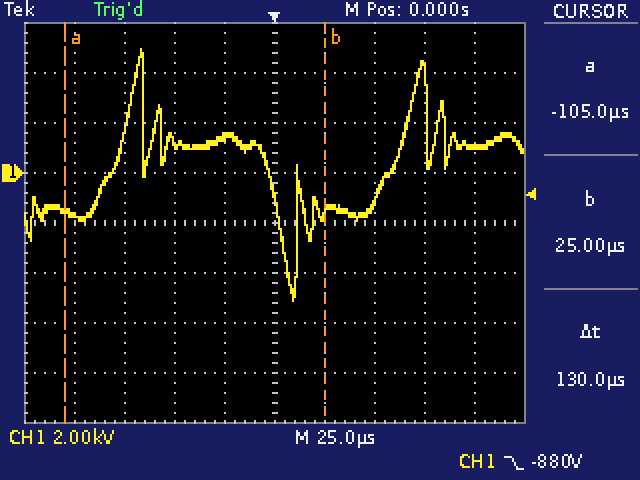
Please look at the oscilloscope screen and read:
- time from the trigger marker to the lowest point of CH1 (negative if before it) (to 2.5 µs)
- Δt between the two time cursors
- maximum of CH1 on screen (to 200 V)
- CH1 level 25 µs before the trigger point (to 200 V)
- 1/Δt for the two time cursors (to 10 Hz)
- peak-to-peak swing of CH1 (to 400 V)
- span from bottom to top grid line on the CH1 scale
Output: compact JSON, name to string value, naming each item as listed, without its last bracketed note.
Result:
{"time from the trigger marker to the lowest point of CH1 (negative if before it)": "+10.0 µs", "Δt between the two time cursors": "130 µs", "maximum of CH1 on screen": "5.0 kV", "CH1 level 25 µs before the trigger point": "1.4 kV", "1/Δt for the two time cursors": "7.69 kHz", "peak-to-peak swing of CH1": "10.0 kV", "span from bottom to top grid line on the CH1 scale": "16 kV"}
